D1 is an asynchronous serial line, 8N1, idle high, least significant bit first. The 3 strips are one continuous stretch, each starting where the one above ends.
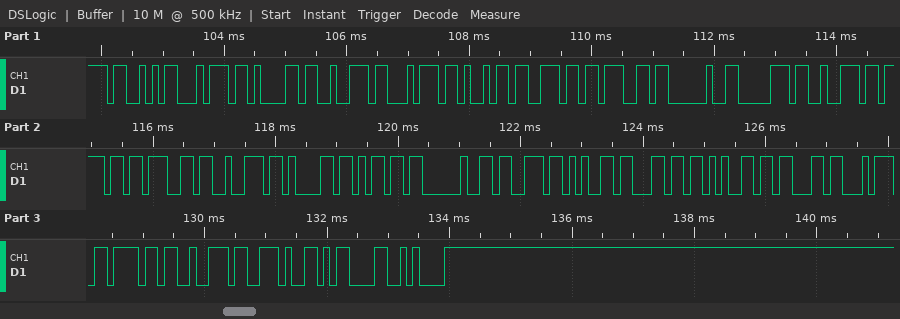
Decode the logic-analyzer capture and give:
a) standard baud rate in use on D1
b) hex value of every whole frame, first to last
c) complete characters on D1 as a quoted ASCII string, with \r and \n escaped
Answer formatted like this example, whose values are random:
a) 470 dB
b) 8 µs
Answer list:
a) 9600 baud
b) 53 74 61 72 74 69 6E 67 20 70 72 6F 67 72 61 6D 20 73 65 6C 65 63 74 6F 72 2E 0D 0A
c) "Starting program selector.\r\n"
